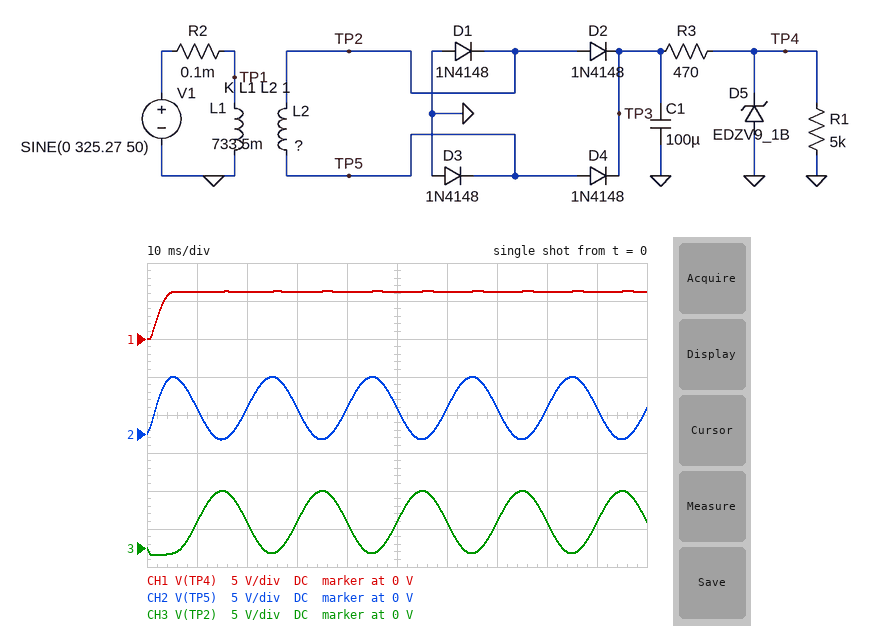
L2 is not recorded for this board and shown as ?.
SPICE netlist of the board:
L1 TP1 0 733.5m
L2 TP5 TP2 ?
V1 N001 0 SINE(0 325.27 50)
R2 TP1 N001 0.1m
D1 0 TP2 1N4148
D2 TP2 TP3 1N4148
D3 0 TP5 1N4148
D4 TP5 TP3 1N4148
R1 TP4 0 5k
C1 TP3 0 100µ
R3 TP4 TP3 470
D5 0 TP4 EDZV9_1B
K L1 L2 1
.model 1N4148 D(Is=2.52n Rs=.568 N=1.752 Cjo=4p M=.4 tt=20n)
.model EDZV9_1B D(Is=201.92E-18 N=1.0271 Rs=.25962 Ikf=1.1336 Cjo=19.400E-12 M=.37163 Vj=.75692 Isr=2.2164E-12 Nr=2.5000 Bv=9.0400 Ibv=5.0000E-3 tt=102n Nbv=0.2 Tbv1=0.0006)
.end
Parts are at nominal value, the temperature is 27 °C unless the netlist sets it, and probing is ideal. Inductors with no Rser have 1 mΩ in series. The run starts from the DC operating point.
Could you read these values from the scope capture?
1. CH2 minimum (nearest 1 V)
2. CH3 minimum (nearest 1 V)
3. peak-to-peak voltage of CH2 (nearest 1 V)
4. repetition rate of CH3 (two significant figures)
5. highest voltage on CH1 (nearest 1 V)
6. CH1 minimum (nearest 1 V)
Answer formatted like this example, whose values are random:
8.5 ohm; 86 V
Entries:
-1 V; -1 V; 8 V; 50 Hz; 6 V; 0 V
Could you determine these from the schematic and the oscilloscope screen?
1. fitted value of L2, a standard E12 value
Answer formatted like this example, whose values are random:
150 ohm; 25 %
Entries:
470 µH
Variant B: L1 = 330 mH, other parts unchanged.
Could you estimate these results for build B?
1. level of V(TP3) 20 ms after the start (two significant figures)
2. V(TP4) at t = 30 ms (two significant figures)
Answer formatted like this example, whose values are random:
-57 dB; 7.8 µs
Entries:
11 V; 9.0 V
